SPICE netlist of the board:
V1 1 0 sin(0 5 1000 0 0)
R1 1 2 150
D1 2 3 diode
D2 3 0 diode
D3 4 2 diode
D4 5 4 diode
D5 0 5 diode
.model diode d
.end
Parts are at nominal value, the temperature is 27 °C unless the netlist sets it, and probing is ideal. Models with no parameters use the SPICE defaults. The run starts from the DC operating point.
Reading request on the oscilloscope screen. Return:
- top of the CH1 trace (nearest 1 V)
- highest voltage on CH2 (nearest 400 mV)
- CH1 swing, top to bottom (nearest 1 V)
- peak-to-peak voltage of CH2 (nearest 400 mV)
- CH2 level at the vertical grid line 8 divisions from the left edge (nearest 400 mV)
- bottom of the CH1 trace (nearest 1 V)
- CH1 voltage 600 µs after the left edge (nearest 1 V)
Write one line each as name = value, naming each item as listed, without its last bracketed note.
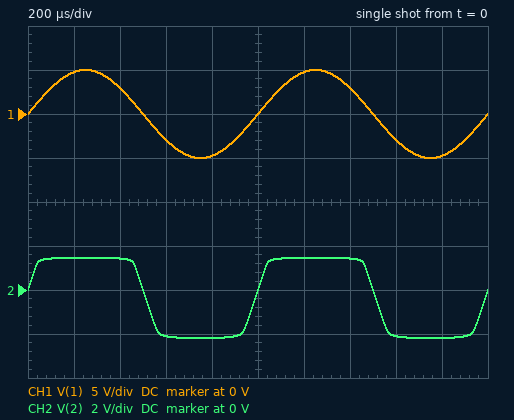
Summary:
top of the CH1 trace = 5 V
highest voltage on CH2 = 1.6 V
CH1 swing, top to bottom = 10 V
peak-to-peak voltage of CH2 = 3.6 V
CH2 level at the vertical grid line 8 divisions from the left edge = -2.0 V
bottom of the CH1 trace = -5 V
CH1 voltage 600 µs after the left edge = -3 V
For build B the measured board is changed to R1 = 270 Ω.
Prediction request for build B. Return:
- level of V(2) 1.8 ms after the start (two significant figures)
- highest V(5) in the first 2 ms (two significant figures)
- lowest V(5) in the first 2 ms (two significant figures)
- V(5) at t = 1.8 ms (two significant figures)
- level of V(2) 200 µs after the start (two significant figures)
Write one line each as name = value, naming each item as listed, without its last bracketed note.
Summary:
level of V(2) 1.8 ms after the start = -2.1 V
highest V(5) in the first 2 ms = 480 mV
lowest V(5) in the first 2 ms = -720 mV
V(5) at t = 1.8 ms = -710 mV
level of V(2) 200 µs after the start = 1.4 V
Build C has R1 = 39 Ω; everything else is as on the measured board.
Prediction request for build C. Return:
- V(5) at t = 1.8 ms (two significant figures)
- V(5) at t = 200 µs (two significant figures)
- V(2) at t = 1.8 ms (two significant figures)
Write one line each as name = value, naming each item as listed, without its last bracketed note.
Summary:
V(5) at t = 1.8 ms = -760 mV
V(5) at t = 200 µs = 510 mV
V(2) at t = 1.8 ms = -2.3 V
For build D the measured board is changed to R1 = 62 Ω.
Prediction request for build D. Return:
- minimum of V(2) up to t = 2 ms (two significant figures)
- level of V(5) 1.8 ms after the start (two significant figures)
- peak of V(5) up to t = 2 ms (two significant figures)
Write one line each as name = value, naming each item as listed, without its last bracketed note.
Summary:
minimum of V(2) up to t = 2 ms = -2.3 V
level of V(5) 1.8 ms after the start = -750 mV
peak of V(5) up to t = 2 ms = 510 mV
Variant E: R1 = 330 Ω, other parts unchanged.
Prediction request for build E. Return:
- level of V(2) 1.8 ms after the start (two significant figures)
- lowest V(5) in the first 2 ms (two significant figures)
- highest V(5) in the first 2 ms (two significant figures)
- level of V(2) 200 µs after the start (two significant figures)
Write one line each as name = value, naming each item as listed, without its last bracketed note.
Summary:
level of V(2) 1.8 ms after the start = -2.1 V
lowest V(5) in the first 2 ms = -710 mV
highest V(5) in the first 2 ms = 480 mV
level of V(2) 200 µs after the start = 1.4 V
